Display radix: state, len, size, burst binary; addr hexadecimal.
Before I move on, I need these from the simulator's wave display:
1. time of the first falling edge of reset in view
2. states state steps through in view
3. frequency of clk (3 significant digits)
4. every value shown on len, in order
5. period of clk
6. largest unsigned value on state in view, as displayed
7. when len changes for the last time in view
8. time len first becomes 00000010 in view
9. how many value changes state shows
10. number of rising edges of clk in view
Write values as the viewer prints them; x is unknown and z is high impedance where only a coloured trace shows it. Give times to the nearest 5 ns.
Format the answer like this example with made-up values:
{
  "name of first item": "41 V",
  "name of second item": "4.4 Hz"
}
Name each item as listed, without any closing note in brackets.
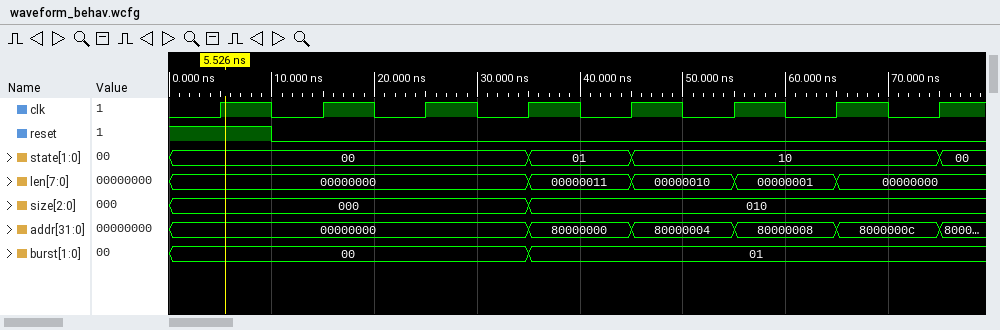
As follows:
{
  "time of the first falling edge of reset in view": "10 ns",
  "states state steps through in view": "00, 01, 10, 00",
  "frequency of clk": "100 MHz",
  "every value shown on len, in order": "00000000, 00000011, 00000010, 00000001, 00000000",
  "period of clk": "10 ns",
  "largest unsigned value on state in view, as displayed": "10",
  "when len changes for the last time in view": "65 ns",
  "time len first becomes 00000010 in view": "45 ns",
  "how many value changes state shows": "3",
  "number of rising edges of clk in view": "8"
}
